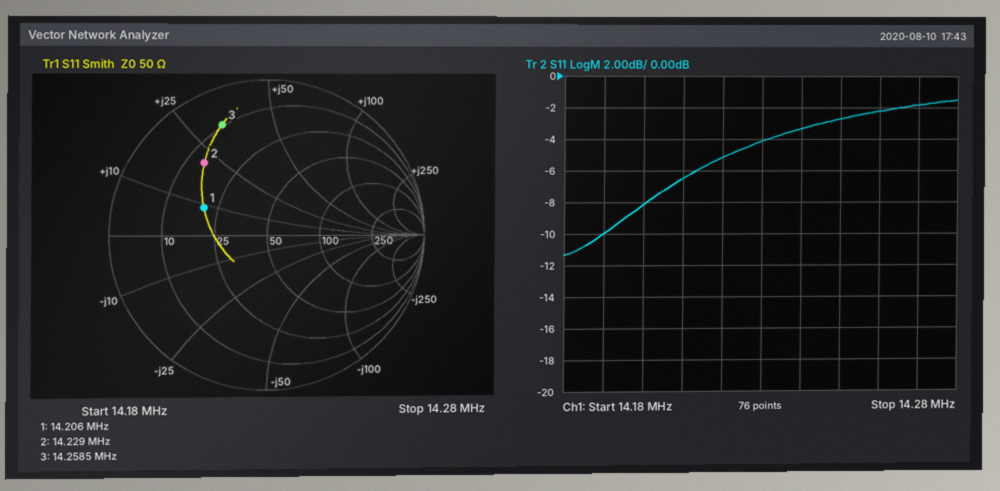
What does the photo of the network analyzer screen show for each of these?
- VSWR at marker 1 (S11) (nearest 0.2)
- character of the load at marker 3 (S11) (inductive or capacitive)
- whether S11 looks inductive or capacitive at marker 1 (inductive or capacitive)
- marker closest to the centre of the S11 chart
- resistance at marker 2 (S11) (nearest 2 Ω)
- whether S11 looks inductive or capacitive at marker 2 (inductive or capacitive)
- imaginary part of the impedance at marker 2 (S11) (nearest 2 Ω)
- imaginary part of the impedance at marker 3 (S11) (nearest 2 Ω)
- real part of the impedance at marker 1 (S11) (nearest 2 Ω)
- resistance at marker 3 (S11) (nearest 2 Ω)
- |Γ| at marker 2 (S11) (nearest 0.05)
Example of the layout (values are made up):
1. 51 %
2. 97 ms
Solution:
1. 2.6
2. inductive
3. inductive
4. marker 1
5. 14 Ω
6. inductive
7. +22 Ω
8. +32 Ω
9. 20 Ω
10. 10 Ω
11. 0.60
